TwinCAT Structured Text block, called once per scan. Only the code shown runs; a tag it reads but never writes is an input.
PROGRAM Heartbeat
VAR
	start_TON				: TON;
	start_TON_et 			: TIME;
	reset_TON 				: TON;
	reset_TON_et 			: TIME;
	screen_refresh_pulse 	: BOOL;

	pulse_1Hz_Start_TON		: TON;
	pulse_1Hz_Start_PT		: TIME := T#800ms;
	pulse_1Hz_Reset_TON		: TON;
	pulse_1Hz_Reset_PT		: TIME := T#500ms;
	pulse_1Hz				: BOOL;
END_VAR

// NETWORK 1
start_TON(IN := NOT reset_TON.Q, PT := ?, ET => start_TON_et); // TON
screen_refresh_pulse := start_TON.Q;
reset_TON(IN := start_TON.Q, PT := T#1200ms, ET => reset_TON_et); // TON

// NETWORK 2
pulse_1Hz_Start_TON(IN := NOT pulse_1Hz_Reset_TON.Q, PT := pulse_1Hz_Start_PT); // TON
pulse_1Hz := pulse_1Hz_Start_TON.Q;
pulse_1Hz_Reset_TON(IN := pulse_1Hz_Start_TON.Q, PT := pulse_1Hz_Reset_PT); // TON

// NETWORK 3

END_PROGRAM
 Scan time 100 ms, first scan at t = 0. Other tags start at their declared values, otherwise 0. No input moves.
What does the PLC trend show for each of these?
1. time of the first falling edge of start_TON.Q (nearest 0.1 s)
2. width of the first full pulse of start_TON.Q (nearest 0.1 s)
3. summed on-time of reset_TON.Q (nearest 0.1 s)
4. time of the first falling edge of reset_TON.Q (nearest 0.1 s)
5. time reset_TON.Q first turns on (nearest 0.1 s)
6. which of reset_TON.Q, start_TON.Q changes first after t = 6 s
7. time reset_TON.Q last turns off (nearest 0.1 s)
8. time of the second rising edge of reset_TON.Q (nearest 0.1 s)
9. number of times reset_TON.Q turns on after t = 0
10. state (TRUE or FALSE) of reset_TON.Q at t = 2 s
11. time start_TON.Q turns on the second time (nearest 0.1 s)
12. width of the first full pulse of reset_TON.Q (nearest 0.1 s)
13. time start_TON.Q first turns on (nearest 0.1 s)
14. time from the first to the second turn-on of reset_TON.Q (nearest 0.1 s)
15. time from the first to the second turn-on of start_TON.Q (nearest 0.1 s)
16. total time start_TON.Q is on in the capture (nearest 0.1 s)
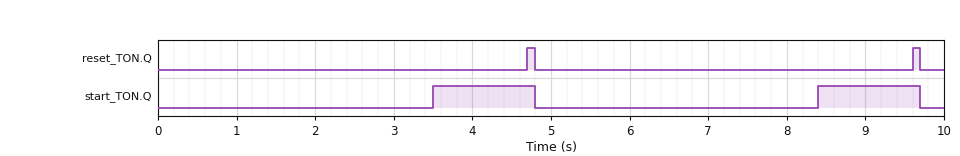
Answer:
4.8 s
1.3 s
0.2 s
4.8 s
4.7 s
start_TON.Q
9.7 s
9.6 s
2
FALSE
8.4 s
0.1 s
3.5 s
4.9 s
4.9 s
2.6 s
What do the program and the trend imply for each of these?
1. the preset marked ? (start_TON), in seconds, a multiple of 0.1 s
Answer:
3.5 s
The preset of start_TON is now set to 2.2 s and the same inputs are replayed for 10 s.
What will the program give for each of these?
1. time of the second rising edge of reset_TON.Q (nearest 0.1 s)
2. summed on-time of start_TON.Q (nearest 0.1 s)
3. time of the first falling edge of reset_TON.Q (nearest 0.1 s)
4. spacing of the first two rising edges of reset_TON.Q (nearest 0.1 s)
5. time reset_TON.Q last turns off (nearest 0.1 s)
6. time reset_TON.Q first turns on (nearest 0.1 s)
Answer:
7.0 s
3.2 s
3.5 s
3.6 s
7.1 s
3.4 s
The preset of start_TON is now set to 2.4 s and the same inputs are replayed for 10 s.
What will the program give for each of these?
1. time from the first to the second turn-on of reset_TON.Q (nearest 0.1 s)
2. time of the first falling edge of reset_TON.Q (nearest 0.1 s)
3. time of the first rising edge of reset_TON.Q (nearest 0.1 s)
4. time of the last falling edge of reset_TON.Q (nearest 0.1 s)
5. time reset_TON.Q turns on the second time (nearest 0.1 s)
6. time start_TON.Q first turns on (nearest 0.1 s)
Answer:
3.8 s
3.7 s
3.6 s
7.5 s
7.4 s
2.4 s
